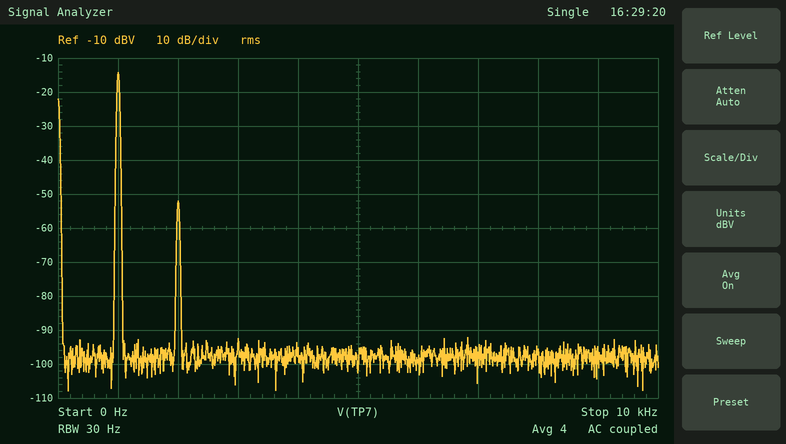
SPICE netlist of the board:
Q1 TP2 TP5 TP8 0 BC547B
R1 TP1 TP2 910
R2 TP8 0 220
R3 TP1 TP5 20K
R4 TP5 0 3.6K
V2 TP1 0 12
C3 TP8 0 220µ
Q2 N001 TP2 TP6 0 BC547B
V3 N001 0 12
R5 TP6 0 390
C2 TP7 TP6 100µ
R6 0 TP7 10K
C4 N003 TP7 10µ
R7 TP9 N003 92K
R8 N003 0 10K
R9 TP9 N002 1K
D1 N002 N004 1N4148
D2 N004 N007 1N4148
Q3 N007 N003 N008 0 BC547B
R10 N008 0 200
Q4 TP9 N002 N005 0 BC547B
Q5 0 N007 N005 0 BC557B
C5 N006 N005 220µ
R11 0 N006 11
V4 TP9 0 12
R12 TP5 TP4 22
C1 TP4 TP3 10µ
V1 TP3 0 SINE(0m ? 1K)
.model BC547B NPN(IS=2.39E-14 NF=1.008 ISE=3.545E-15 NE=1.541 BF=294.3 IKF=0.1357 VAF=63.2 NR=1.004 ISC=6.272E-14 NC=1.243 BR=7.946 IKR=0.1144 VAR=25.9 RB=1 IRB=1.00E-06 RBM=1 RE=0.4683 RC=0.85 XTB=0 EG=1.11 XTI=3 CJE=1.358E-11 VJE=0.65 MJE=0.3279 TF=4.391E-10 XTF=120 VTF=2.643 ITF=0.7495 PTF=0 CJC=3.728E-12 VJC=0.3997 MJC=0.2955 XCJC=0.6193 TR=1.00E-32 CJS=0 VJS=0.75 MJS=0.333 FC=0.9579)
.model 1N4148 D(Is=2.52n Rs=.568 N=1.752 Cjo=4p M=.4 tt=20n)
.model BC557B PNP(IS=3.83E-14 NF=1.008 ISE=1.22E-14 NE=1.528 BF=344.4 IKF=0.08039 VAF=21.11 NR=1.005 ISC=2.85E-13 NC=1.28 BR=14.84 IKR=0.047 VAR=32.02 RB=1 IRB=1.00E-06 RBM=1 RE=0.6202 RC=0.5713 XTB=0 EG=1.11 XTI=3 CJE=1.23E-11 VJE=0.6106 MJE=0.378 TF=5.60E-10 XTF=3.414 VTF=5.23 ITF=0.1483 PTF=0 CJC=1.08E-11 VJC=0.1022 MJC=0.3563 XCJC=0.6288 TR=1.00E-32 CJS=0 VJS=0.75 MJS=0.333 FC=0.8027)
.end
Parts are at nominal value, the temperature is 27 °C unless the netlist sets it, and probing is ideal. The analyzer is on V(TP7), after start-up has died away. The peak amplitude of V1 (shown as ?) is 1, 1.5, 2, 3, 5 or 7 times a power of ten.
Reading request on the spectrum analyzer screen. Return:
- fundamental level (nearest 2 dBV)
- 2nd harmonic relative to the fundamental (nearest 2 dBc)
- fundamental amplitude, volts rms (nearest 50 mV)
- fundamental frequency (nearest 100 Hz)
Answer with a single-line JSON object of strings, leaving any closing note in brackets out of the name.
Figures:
{"fundamental level": "-14 dBV", "2nd harmonic relative to the fundamental": "-38 dBc", "fundamental amplitude, volts rms": "200 mV", "fundamental frequency": "1.0 kHz"}
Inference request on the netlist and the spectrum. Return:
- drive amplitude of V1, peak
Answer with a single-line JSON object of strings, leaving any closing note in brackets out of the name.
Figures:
{"drive amplitude of V1, peak": "2 mV"}
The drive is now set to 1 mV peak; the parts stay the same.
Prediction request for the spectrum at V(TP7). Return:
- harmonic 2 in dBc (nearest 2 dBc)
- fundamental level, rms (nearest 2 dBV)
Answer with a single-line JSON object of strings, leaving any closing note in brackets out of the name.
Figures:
{"harmonic 2 in dBc": "-44 dBc", "fundamental level, rms": "-20 dBV"}
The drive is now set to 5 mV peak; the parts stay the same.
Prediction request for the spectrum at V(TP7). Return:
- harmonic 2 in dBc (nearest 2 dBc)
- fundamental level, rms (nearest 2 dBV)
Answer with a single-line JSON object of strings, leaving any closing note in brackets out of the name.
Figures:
{"harmonic 2 in dBc": "-30 dBc", "fundamental level, rms": "-6 dBV"}
